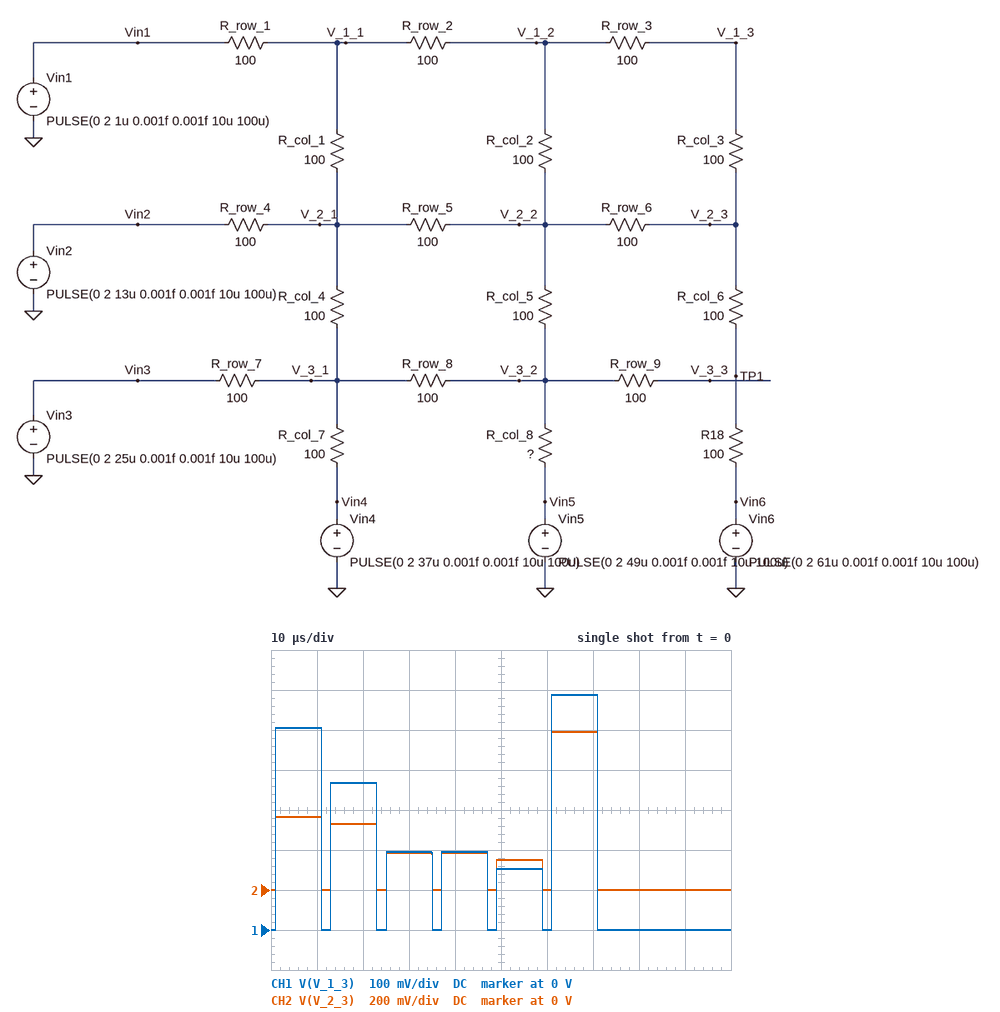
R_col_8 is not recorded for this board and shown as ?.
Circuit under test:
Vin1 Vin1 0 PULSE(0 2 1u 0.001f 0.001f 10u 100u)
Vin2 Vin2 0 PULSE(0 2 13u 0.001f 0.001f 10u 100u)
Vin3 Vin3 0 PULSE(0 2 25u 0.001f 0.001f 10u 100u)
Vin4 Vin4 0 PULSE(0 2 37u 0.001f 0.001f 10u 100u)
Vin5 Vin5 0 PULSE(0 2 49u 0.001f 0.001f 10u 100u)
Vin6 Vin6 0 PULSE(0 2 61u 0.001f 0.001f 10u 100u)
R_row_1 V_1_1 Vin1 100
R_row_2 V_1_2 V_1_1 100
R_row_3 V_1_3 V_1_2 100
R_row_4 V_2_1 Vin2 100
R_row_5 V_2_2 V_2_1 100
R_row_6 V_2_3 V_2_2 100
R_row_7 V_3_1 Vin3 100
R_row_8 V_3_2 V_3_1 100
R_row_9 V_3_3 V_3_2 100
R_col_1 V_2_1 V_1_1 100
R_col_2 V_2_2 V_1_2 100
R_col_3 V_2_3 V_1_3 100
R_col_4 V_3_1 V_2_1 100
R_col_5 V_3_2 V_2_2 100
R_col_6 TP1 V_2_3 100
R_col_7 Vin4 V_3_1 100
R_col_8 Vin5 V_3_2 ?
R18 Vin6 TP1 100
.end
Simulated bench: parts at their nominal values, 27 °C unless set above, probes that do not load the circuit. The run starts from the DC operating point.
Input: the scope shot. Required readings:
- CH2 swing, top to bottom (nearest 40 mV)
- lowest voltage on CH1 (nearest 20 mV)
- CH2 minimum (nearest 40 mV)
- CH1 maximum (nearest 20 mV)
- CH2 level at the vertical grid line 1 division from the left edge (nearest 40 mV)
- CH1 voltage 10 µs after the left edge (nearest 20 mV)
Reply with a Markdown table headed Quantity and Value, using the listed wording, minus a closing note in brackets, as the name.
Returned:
| Quantity | Value |
|---|---|
| CH2 swing, top to bottom | 800 mV |
| lowest voltage on CH1 | 0 V |
| CH2 minimum | 0 V |
| CH1 maximum | 580 mV |
| CH2 level at the vertical grid line 1 division from the left edge | 360 mV |
| CH1 voltage 10 µs after the left edge | 500 mV |
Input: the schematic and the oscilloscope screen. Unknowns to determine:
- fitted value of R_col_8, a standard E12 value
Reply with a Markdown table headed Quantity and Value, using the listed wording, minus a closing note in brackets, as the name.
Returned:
| Quantity | Value |
|---|---|
| fitted value of R_col_8, a standard E12 value | 270 Ω |
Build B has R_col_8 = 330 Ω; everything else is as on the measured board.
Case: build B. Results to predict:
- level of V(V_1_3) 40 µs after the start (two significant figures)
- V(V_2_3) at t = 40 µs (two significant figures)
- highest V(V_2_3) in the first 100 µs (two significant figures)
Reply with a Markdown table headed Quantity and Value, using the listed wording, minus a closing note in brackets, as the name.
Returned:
| Quantity | Value |
|---|---|
| level of V(V_1_3) 40 µs after the start | 200 mV |
| V(V_2_3) at t = 40 µs | 190 mV |
| highest V(V_2_3) in the first 100 µs | 790 mV |
